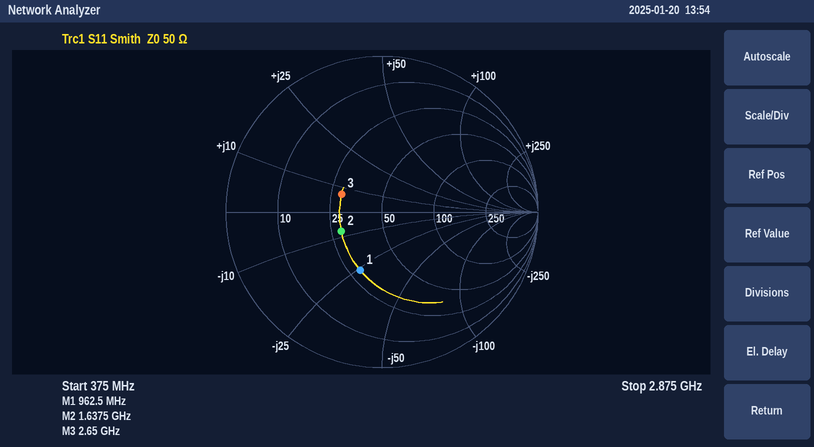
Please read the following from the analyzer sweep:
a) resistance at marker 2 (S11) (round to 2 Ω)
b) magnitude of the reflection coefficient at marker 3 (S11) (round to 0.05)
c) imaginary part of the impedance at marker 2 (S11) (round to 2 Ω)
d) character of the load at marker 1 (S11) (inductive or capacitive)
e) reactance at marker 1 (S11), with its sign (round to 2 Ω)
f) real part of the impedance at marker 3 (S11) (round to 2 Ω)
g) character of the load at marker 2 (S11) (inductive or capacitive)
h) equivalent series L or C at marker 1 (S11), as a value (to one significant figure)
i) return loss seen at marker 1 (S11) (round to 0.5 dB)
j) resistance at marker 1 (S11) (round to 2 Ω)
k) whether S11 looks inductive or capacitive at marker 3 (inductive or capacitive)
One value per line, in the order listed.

28 Ω
0.30
-8 Ω
capacitive
-26 Ω
28 Ω
capacitive
6 pF
8.0 dB
30 Ω
inductive
